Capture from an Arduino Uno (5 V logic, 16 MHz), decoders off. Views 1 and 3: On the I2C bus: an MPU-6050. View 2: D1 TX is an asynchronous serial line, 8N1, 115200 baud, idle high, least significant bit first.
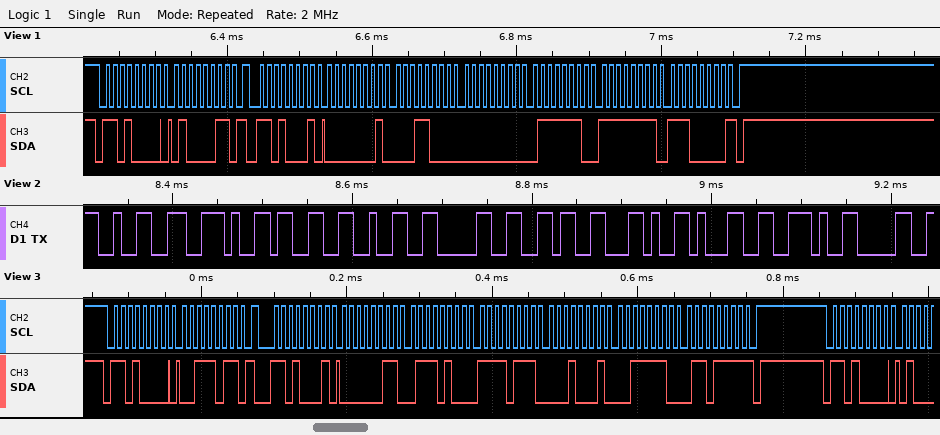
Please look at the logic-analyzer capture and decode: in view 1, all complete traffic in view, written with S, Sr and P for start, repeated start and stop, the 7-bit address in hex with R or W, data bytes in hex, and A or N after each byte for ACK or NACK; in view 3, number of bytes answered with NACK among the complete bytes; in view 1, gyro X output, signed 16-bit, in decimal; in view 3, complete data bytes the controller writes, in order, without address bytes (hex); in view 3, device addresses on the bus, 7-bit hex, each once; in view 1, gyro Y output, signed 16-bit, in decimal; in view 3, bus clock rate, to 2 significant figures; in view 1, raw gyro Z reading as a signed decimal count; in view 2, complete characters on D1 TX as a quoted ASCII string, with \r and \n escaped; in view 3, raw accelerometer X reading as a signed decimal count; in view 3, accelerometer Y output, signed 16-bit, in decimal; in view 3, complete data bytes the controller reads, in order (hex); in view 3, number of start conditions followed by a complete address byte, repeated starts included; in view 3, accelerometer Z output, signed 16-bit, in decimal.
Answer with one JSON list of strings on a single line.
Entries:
["S 68W A 43 A Sr 68R A 01 A 18 A 00 A 7E A FF A E0 N P", "1", "280", "3B", "0x68", "126", "100 kHz", "-32", "\"2.3206,1.0\"", "884", "-2287", "03 74 F7 11 3E 6F", "3", "15983"]
